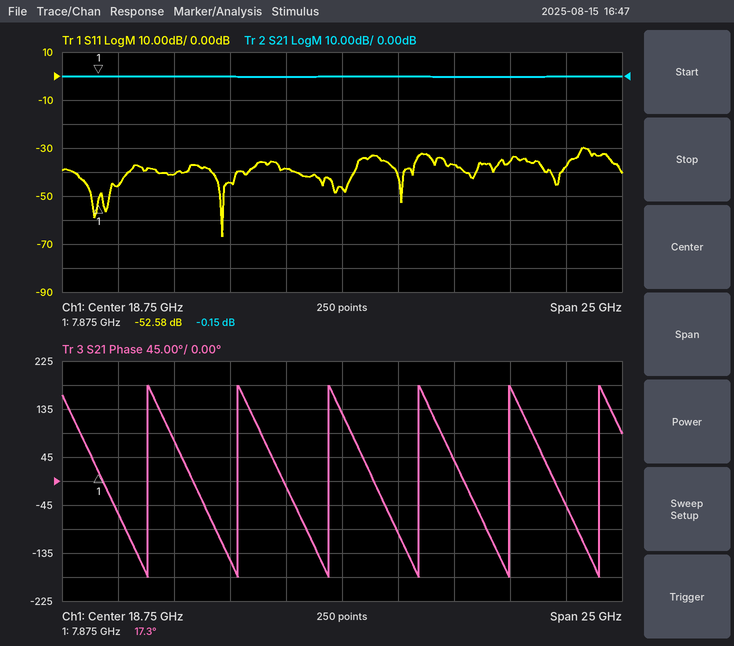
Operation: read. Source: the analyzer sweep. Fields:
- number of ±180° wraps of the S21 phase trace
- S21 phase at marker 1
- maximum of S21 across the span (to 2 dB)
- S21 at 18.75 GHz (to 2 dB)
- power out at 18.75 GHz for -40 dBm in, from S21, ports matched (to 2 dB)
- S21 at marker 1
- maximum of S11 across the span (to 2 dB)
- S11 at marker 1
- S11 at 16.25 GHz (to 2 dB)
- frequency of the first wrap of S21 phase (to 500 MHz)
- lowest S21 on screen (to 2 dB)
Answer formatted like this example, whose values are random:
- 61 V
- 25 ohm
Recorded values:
- 6
- 17.3°
- 0 dB
- 0 dB
- -40 dBm
- -0.15 dB
- -30 dB
- -52.58 dB
- -38 dB
- 10.0 GHz
- 0 dB
